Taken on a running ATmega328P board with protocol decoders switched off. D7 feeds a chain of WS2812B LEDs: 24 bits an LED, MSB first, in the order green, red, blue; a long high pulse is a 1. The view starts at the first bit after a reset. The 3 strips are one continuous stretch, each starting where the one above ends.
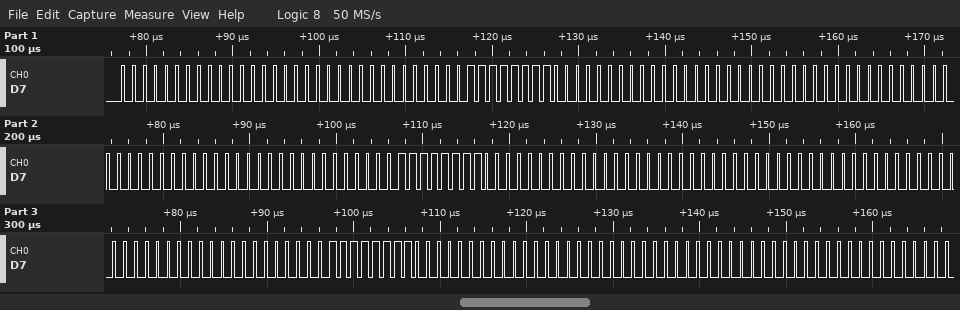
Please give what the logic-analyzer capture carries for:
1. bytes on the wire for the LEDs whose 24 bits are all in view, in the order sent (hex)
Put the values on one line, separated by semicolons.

00 00 00 00 FF 00 00 00 00 00 00 00 00 FF 00 00 00 00 00 00 00 00 FF 00 00 00 00
